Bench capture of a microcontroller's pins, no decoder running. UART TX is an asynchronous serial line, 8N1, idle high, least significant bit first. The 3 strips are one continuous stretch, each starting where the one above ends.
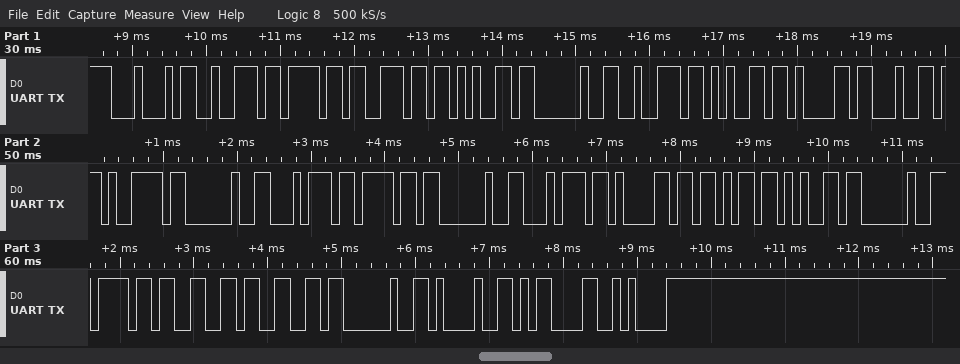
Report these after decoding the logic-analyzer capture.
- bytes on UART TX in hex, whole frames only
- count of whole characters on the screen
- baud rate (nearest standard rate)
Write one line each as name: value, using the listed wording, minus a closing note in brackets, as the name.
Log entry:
bytes on UART TX in hex, whole frames only: 44 72 6F 6E 65 20 72 65 61 64 79 20 74 6F 20 74 61 6B 65 20 6F 66 66 20 21 0D 0A
count of whole characters on the screen: 27
baud rate: 9600 baud
